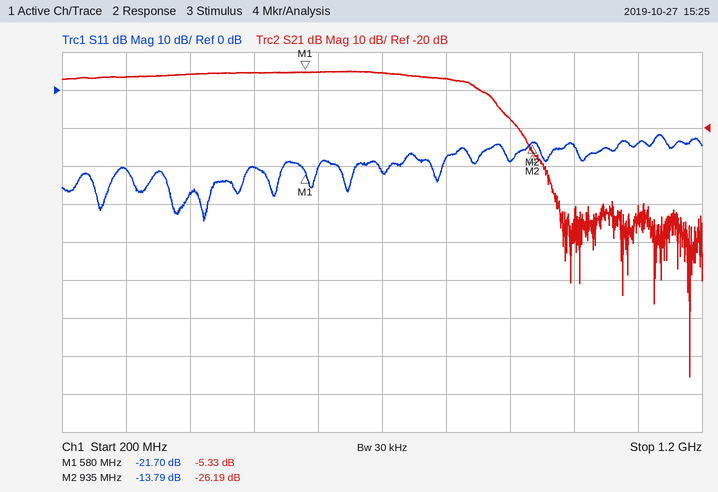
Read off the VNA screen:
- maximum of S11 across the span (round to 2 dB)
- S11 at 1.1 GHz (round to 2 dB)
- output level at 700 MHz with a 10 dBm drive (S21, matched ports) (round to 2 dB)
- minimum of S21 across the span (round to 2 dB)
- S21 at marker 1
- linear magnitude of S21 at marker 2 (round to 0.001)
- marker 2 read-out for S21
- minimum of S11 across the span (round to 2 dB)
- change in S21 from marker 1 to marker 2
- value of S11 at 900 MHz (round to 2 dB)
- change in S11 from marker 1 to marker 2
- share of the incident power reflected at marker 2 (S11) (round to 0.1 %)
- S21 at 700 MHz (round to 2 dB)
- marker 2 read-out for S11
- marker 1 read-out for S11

-12 dB
-14 dB
4 dBm
-86 dB
-5.33 dB
0.049
-26.19 dB
-34 dB
-20.86 dB
-18 dB
7.91 dB
4.2 %
-6 dB
-13.79 dB
-21.70 dB
